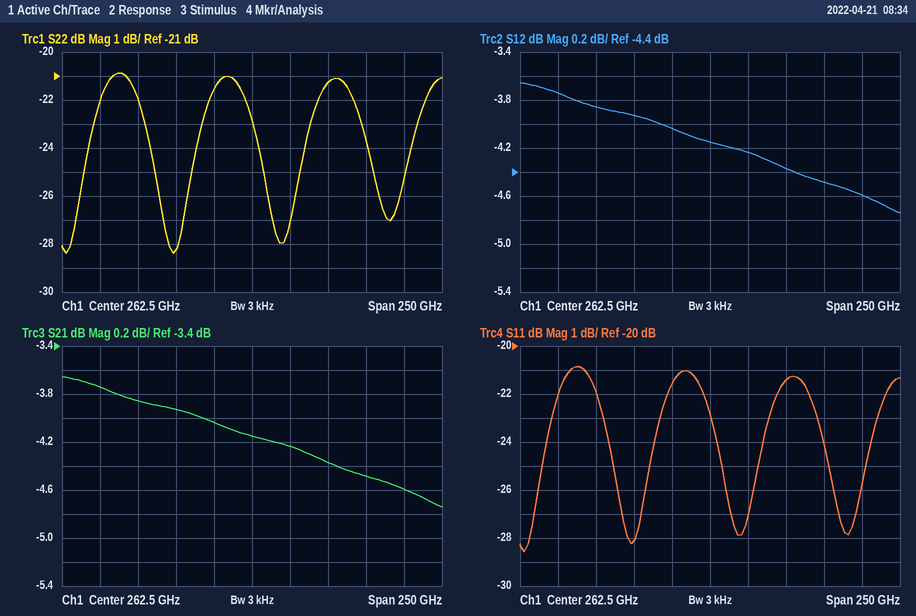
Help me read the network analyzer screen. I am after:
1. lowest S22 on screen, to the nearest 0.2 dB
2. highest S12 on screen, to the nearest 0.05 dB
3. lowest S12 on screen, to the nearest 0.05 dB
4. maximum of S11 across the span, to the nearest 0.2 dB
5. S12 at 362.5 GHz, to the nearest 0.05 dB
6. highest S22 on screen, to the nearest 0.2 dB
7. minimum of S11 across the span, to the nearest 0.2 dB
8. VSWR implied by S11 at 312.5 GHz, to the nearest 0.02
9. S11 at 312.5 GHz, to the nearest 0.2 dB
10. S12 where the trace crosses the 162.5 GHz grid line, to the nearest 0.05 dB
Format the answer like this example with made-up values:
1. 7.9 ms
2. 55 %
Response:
1. -28.4 dB
2. -3.65 dB
3. -4.75 dB
4. -20.8 dB
5. -4.60 dB
6. -20.8 dB
7. -28.6 dB
8. 1.18
9. -21.4 dB
10. -3.75 dB
